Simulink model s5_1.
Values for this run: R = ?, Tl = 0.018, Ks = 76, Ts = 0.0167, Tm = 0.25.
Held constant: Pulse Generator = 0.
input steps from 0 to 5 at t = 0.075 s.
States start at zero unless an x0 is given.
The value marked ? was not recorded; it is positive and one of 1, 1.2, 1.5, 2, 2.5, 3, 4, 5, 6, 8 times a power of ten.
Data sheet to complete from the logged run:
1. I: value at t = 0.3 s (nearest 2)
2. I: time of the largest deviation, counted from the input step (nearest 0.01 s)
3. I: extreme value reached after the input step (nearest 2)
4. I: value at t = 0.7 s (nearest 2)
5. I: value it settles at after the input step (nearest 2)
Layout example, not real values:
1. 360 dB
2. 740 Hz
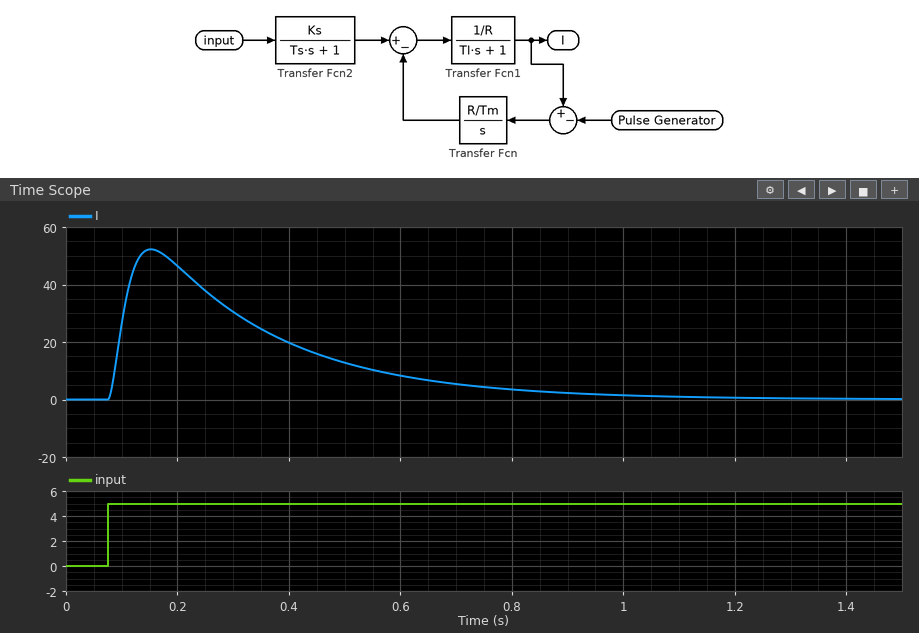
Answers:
1. 30
2. 0.08 s
3. 52
4. 6
5. 0
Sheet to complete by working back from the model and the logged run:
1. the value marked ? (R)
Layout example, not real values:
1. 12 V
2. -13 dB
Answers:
1. 6
